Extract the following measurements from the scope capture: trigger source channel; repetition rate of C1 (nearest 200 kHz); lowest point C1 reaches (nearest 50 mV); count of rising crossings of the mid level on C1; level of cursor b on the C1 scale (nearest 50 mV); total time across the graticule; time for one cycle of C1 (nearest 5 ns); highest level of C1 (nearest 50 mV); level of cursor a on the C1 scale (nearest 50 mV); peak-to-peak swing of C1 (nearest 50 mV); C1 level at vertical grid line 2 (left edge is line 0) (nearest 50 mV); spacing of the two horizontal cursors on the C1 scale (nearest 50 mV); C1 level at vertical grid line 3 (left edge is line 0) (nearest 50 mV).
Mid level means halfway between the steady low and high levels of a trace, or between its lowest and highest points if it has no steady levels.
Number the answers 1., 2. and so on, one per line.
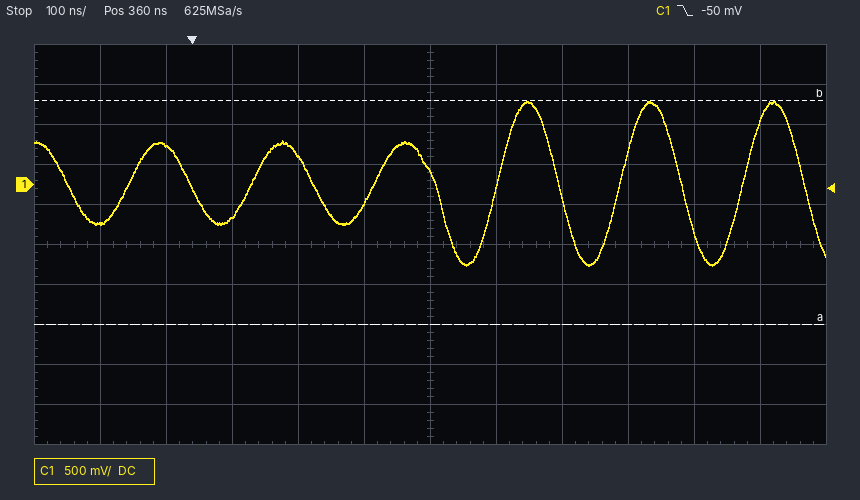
1. C1
2. 5.4 MHz
3. -1.00 V
4. 6
5. 1.05 V
6. 1.2 µs
7. 185 ns
8. 1.05 V
9. -1.75 V
10. 2.05 V
11. 500 mV
12. 2.80 V
13. -400 mV
